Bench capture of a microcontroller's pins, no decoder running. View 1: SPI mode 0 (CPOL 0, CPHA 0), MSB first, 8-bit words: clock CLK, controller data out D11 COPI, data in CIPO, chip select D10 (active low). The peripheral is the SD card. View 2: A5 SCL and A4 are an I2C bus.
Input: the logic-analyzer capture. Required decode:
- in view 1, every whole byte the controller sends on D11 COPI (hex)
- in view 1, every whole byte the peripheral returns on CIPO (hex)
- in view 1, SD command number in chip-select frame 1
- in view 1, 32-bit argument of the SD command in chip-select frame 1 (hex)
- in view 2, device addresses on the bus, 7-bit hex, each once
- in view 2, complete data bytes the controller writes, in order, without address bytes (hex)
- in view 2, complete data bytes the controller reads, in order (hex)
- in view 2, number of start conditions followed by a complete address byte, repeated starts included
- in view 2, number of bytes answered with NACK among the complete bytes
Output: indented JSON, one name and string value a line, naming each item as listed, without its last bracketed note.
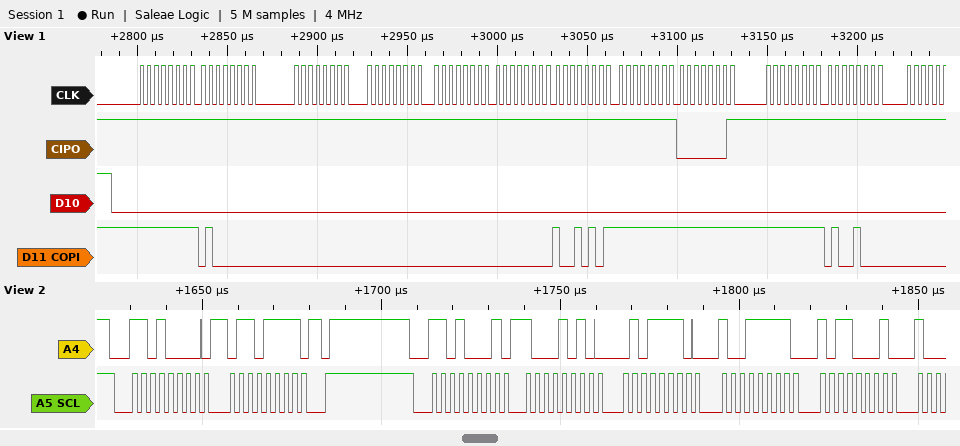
{
  "in view 1, every whole byte the controller sends on D11 COPI": "FF 40 00 00 00 00 95 FF FF FF 48",
  "in view 1, every whole byte the peripheral returns on CIPO": "FF FF FF FF FF FF FF FF 01 FF FF",
  "in view 1, SD command number in chip-select frame 1": "CMD0",
  "in view 1, 32-bit argument of the SD command in chip-select frame 1": "0x00000000",
  "in view 2, device addresses on the bus, 7-bit hex, each once": "0x68",
  "in view 2, complete data bytes the controller writes, in order, without address bytes": "6F",
  "in view 2, complete data bytes the controller reads, in order": "8A 5E 9F B1",
  "in view 2, number of start conditions followed by a complete address byte, repeated starts included": "2",
  "in view 2, number of bytes answered with NACK among the complete bytes": "0"
}
